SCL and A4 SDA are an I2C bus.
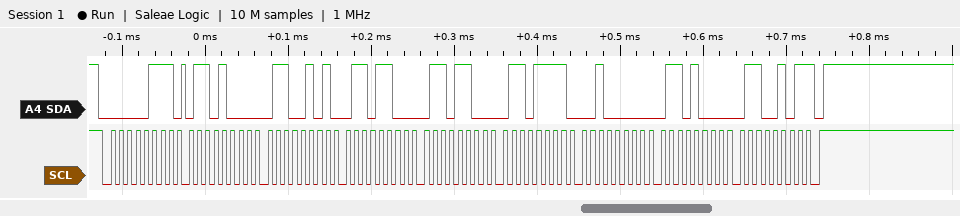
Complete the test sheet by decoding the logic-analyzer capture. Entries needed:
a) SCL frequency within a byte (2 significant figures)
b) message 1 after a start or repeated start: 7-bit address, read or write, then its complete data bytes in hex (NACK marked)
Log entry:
100 kHz
0x03 read: 68 65 6C 6C 6F 20 68 65 NACK
